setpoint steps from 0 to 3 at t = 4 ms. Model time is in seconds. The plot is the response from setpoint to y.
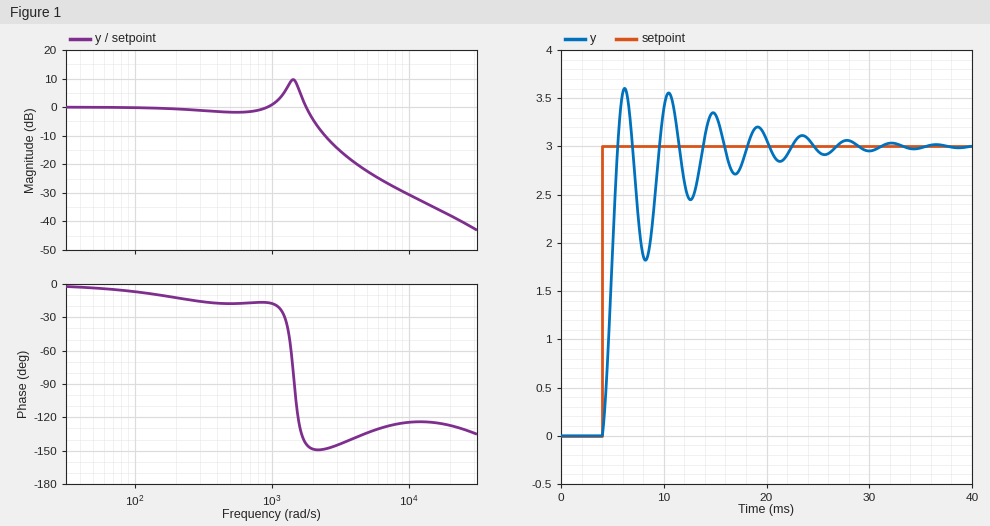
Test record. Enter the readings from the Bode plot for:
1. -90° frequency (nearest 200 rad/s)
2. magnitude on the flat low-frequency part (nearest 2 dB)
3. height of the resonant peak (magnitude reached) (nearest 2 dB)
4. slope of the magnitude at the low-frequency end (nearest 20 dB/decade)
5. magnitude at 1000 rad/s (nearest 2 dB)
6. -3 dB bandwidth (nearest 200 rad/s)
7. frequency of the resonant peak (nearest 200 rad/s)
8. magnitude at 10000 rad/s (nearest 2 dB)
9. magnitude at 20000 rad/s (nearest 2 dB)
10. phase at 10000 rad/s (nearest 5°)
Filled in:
1400 rad/s
0 dB
10 dB
0 dB/decade
0 dB
2000 rad/s
1400 rad/s
-30 dB
-38 dB
-125°
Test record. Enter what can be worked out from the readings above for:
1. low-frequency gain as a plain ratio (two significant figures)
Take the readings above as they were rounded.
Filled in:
1.0
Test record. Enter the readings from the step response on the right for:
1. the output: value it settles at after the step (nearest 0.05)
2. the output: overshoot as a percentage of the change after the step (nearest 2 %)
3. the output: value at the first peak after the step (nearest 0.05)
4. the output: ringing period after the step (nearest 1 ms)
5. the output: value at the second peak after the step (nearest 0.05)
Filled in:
3.00
20 %
3.60
4 ms
3.55
